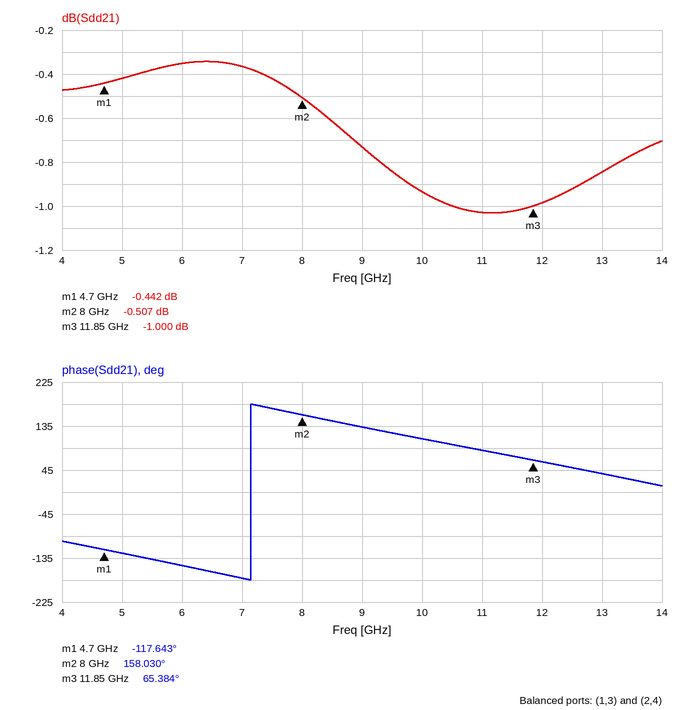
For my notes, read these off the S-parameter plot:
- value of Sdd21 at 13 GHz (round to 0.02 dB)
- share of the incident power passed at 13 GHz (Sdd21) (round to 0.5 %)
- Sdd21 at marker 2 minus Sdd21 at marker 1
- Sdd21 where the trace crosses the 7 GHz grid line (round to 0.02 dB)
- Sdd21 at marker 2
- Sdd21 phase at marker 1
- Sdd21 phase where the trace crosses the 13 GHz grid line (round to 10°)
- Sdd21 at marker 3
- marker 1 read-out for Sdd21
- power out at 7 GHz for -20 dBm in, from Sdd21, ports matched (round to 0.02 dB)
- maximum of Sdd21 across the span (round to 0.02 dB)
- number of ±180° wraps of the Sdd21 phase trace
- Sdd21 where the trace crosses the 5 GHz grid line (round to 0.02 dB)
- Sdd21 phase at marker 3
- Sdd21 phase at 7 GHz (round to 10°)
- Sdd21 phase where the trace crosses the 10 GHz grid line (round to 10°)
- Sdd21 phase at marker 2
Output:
-0.84 dB
82.5 %
-0.065 dB
-0.36 dB
-0.507 dB
-117.643°
40°
-1.000 dB
-0.442 dB
-20.36 dBm
-0.34 dB
1
-0.42 dB
65.384°
-180°
110°
158.030°
